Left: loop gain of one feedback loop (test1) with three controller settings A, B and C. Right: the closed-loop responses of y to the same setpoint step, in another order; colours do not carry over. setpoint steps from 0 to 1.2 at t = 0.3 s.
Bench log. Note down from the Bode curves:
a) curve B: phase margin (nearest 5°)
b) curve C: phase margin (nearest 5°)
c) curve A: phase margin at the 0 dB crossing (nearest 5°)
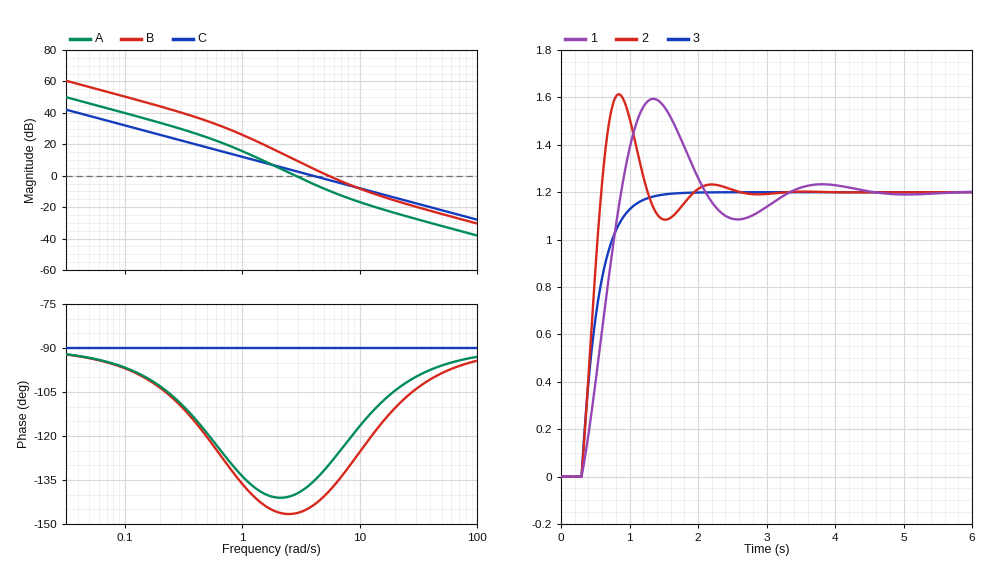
40°
90°
40°
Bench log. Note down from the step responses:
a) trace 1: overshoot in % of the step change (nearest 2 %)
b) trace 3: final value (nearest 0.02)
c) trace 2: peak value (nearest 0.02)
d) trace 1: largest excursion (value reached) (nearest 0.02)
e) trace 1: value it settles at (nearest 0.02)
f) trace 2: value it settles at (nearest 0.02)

32 %
1.20
1.62
1.60
1.20
1.20
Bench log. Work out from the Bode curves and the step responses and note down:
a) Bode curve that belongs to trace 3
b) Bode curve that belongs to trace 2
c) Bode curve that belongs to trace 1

C
B
A
